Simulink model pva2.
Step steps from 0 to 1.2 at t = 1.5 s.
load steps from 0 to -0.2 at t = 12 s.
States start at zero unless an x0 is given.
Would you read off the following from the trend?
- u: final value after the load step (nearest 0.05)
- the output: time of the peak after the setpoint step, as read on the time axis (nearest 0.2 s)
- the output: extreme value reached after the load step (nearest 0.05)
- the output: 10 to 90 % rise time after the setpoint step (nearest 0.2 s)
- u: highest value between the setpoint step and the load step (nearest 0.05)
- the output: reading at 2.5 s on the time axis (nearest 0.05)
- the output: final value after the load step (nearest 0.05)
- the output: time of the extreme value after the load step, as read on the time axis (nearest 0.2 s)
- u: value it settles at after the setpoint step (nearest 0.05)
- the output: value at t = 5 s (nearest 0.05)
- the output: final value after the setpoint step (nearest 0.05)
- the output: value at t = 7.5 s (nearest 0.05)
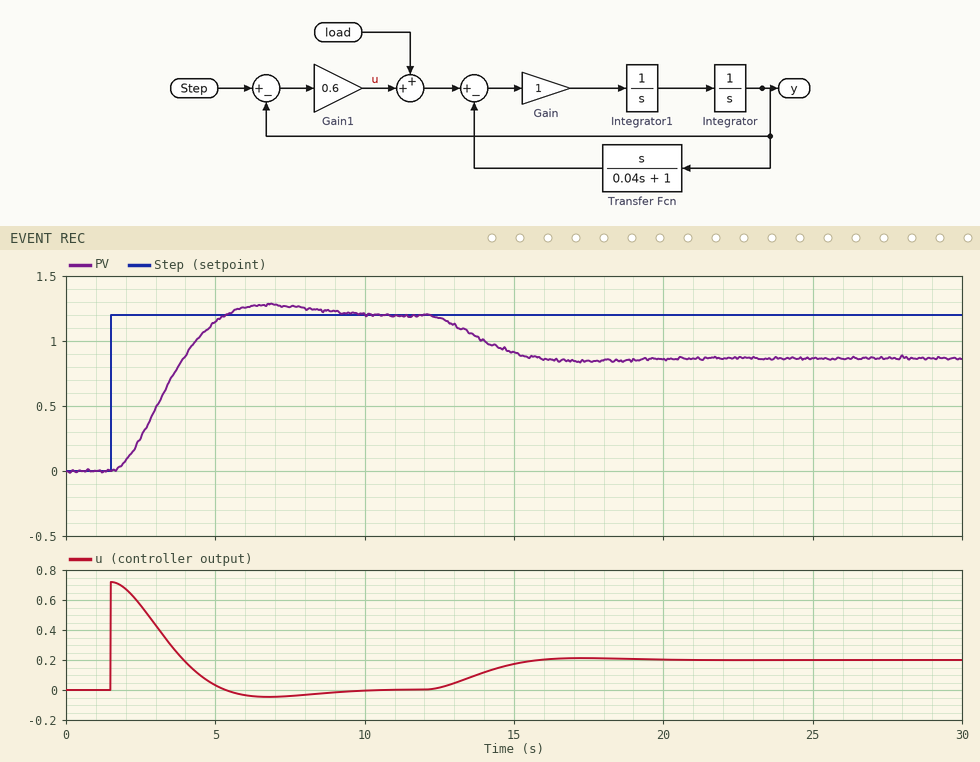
0.20
6.8 s
0.85
2.6 s
0.70
0.25
0.85
17.2 s
0.00
1.15
1.20
1.25
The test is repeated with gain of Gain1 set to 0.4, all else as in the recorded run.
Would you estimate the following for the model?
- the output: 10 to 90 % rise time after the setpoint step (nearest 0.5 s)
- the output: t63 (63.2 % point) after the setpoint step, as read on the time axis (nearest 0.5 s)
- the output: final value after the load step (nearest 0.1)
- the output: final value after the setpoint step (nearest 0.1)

4.0 s
4.5 s
0.7
1.2
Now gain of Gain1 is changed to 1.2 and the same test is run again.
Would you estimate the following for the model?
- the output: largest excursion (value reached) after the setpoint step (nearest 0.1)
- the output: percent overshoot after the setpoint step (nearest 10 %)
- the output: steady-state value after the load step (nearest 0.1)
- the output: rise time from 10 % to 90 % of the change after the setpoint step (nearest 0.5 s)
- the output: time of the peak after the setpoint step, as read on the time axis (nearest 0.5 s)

1.4
20 %
1.0
1.5 s
4.5 s
